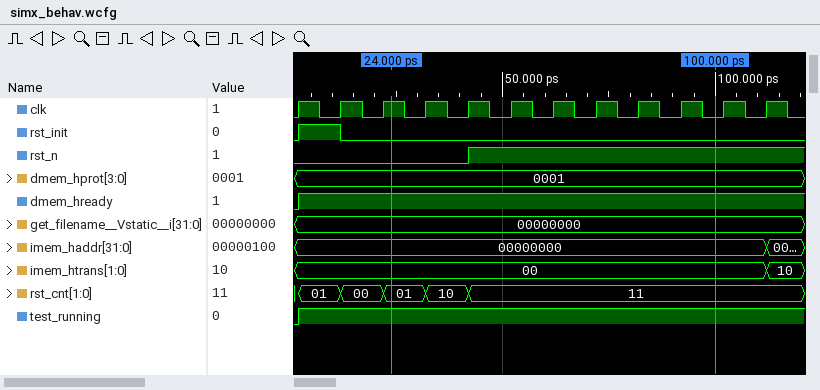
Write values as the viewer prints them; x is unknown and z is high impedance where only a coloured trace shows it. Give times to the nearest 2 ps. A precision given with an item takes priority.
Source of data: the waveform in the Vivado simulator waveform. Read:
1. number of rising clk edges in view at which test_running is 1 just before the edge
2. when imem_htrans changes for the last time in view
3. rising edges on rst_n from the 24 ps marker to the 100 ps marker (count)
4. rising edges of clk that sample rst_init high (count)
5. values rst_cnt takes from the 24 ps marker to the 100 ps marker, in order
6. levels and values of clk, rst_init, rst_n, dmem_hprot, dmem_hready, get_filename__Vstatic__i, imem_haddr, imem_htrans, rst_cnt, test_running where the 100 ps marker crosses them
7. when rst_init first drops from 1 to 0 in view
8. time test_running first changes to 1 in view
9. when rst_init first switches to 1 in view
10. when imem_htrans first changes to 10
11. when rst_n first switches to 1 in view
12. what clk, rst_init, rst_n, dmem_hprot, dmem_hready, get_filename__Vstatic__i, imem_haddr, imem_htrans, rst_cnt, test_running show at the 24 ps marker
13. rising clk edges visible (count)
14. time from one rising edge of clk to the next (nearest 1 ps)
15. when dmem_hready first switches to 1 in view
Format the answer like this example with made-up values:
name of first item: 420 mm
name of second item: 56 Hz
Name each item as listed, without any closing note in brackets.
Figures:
number of rising clk edges in view at which test_running is 1 just before the edge: 11
when imem_htrans changes for the last time in view: 112 ps
rising edges on rst_n from the 24 ps marker to the 100 ps marker: 1
rising edges of clk that sample rst_init high: 1
values rst_cnt takes from the 24 ps marker to the 100 ps marker, in order: 01, 10, 11
levels and values of clk, rst_init, rst_n, dmem_hprot, dmem_hready, get_filename__Vstatic__i, imem_haddr, imem_htrans, rst_cnt, test_running where the 100 ps marker crosses them: clk=0, rst_init=0, rst_n=1, dmem_hprot=0001, dmem_hready=1, get_filename__Vstatic__i=00000000, imem_haddr=00000000, imem_htrans=00, rst_cnt=11, test_running=1
when rst_init first drops from 1 to 0 in view: 12 ps
time test_running first changes to 1 in view: 2 ps
when rst_init first switches to 1 in view: 2 ps
when imem_htrans first changes to 10: 112 ps
when rst_n first switches to 1 in view: 42 ps
what clk, rst_init, rst_n, dmem_hprot, dmem_hready, get_filename__Vstatic__i, imem_haddr, imem_htrans, rst_cnt, test_running show at the 24 ps marker: clk=1, rst_init=0, rst_n=0, dmem_hprot=0001, dmem_hready=1, get_filename__Vstatic__i=00000000, imem_haddr=00000000, imem_htrans=00, rst_cnt=01, test_running=1
rising clk edges visible: 12
time from one rising edge of clk to the next: 10 ps
when dmem_hready first switches to 1 in view: 2 ps
